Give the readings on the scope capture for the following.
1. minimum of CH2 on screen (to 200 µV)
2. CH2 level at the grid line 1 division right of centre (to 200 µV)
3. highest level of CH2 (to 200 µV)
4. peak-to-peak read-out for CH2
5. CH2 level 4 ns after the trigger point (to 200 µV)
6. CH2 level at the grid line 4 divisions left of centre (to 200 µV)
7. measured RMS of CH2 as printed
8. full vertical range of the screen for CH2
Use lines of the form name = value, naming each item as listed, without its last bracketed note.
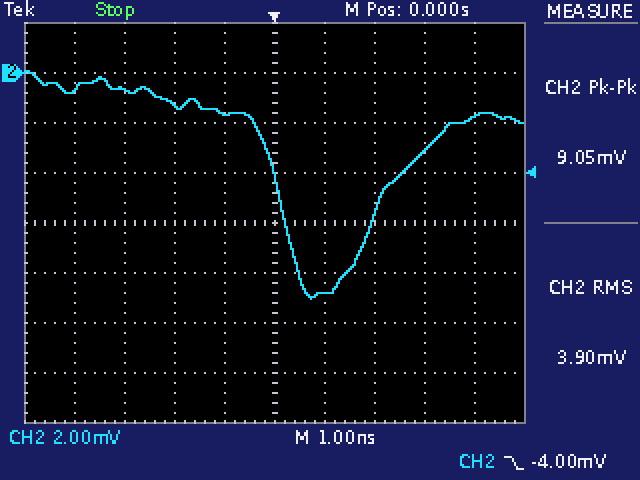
minimum of CH2 on screen = -9.0 mV
CH2 level at the grid line 1 division right of centre = -8.8 mV
highest level of CH2 = 0.0 mV
peak-to-peak read-out for CH2 = 9.05 mV
CH2 level 4 ns after the trigger point = -1.8 mV
CH2 level at the grid line 4 divisions left of centre = -600 µV
measured RMS of CH2 as printed = 3.90 mV
full vertical range of the screen for CH2 = 16 mV
